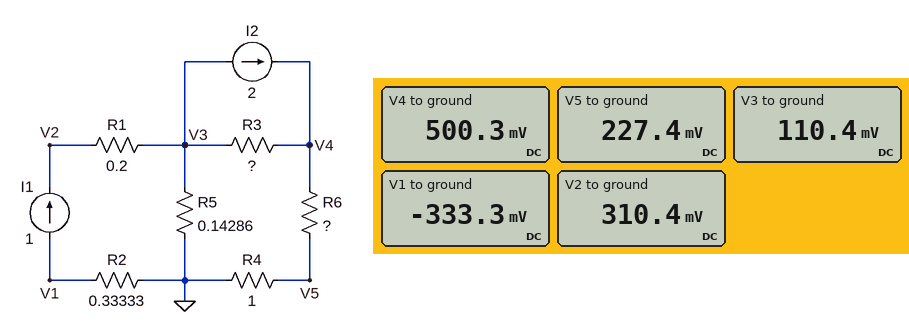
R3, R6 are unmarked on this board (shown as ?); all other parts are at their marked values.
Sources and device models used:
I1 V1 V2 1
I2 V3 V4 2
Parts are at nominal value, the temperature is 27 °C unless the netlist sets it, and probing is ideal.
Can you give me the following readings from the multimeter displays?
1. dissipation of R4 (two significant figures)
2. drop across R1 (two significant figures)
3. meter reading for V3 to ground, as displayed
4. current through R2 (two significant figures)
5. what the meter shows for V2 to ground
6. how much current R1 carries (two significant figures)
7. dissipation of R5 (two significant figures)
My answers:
52 mW
200 mV
110.4 mV
1.0 A
310.4 mV
1.0 A
85 mW
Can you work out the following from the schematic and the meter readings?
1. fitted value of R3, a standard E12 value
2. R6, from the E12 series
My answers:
0.22 Ω
1.2 Ω
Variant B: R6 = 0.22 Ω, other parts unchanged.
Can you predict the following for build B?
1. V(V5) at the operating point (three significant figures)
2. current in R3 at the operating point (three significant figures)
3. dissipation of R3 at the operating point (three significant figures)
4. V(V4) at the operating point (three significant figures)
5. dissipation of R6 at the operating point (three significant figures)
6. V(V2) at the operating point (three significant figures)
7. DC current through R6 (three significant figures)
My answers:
368 mV
1.63 A
586 mW
449 mV
29.8 mW
290 mV
368 mA
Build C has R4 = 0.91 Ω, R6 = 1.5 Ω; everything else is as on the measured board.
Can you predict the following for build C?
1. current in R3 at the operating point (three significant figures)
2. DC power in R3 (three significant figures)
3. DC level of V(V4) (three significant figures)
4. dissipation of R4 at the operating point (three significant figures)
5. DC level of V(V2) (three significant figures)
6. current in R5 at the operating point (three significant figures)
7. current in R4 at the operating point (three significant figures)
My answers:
1.79 A
705 mW
507 mV
40.2 mW
313 mV
790 mA
210 mA
